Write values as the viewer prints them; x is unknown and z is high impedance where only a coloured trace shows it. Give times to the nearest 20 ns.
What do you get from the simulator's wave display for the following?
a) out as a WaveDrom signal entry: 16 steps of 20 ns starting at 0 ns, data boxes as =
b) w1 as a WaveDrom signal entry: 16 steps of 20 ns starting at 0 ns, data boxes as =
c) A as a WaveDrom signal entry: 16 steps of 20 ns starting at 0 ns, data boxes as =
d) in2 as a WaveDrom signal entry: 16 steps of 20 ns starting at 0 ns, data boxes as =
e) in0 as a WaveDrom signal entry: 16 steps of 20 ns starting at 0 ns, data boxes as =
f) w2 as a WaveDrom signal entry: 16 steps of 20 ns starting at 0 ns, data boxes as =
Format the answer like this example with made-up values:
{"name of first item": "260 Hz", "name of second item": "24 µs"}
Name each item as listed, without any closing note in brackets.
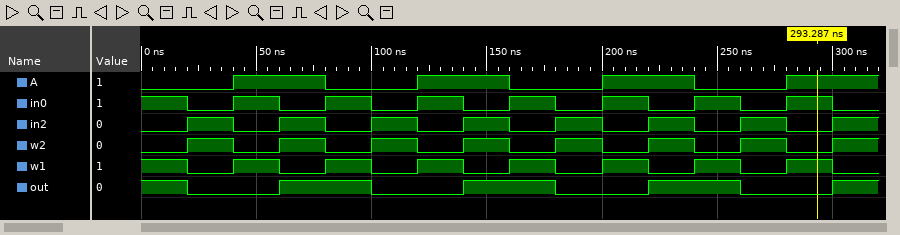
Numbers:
{"out as a WaveDrom signal entry: 16 steps of 20 ns starting at 0 ns, data boxes as =": "{name: 'out', wave: '10.1.0.1.0.1.0.1'}", "w1 as a WaveDrom signal entry: 16 steps of 20 ns starting at 0 ns, data boxes as =": "{name: 'w1', wave: '1010101010101010'}", "A as a WaveDrom signal entry: 16 steps of 20 ns starting at 0 ns, data boxes as =": "{name: 'A', wave: '0.1.0.1.0.1.0.1.'}", "in2 as a WaveDrom signal entry: 16 steps of 20 ns starting at 0 ns, data boxes as =": "{name: 'in2', wave: '0101010101010101'}", "in0 as a WaveDrom signal entry: 16 steps of 20 ns starting at 0 ns, data boxes as =": "{name: 'in0', wave: '1010101010101010'}", "w2 as a WaveDrom signal entry: 16 steps of 20 ns starting at 0 ns, data boxes as =": "{name: 'w2', wave: '0101010101010101'}"}
